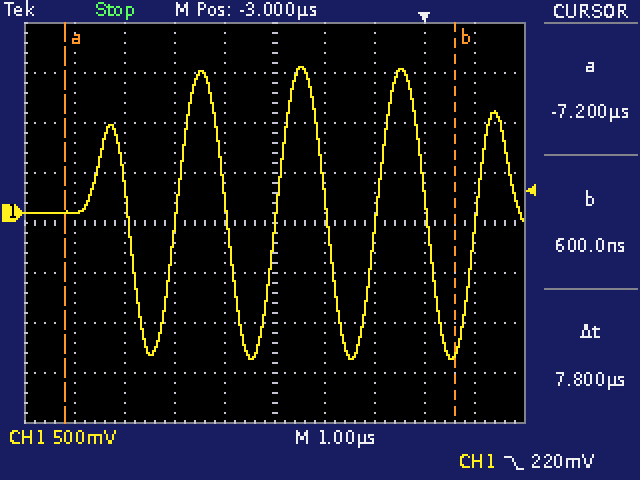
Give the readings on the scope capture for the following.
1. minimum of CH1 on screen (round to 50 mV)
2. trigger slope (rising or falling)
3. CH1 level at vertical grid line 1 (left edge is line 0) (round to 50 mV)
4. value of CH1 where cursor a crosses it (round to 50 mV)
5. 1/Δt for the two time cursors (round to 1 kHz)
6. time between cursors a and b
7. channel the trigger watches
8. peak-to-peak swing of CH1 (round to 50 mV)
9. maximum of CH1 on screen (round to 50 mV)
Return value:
-1.45 V
falling
0 mV
0 mV
128 kHz
7.8 µs
CH1
2.90 V
1.45 V
